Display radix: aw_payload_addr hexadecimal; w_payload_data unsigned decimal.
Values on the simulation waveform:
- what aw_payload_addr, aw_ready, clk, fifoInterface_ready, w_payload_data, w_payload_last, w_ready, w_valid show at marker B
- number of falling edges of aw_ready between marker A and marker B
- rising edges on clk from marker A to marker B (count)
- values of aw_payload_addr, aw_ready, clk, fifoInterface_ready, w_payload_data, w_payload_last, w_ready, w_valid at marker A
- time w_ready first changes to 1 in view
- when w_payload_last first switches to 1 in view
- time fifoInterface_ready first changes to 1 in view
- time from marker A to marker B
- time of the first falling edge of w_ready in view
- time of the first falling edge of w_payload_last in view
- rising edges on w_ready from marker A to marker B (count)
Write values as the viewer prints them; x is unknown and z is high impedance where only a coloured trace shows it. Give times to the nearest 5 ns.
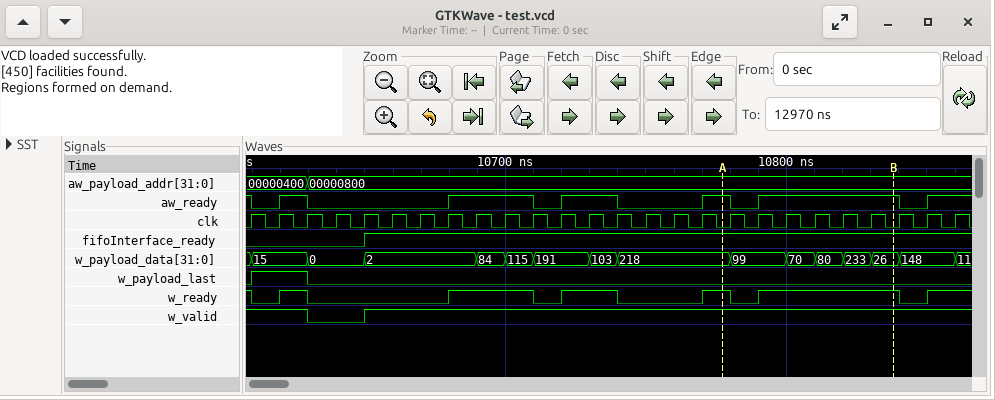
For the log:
aw_payload_addr=00000800, aw_ready=1, clk=0, fifoInterface_ready=1, w_payload_data=26, w_payload_last=0, w_ready=1, w_valid=1
1
6
aw_payload_addr=00000800, aw_ready=1, clk=0, fifoInterface_ready=1, w_payload_data=218, w_payload_last=0, w_ready=1, w_valid=1
10620 ns
10610 ns
10650 ns
60 ns
10610 ns
10630 ns
1
